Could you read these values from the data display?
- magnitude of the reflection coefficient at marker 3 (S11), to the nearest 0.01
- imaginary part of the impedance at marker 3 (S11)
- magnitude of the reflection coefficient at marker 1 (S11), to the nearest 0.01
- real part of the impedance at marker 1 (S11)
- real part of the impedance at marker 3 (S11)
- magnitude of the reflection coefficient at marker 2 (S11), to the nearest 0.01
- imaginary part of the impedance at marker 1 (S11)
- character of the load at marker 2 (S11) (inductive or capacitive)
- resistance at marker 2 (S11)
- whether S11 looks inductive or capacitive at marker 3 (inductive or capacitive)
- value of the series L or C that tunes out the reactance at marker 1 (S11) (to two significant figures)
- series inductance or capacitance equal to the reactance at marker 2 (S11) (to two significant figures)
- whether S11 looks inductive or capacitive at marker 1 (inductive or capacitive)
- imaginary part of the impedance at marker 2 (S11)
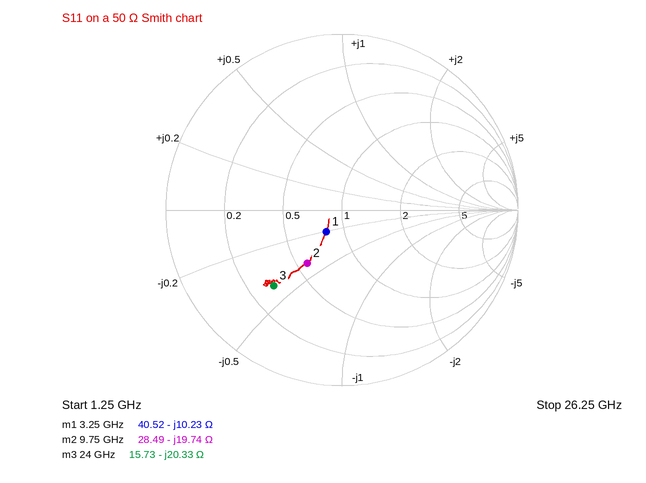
0.58
-20.33 Ω
0.15
40.52 Ω
15.73 Ω
0.36
-10.23 Ω
capacitive
28.49 Ω
capacitive
500 pH
830 fF
capacitive
-19.74 Ω
